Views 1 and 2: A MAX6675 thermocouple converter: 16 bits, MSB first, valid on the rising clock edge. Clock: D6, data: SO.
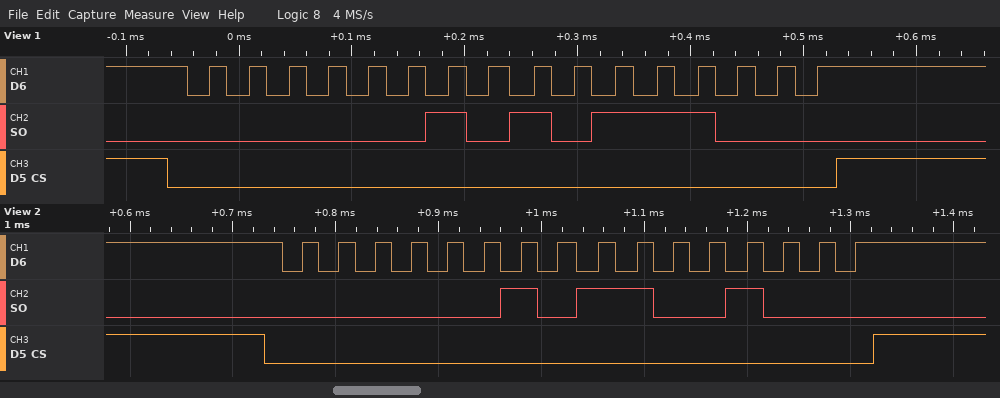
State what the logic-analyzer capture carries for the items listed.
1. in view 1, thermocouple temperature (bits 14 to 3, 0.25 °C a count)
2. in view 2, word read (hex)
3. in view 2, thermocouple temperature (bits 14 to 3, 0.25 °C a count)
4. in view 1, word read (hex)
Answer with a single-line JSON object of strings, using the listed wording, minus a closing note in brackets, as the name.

{"in view 1, thermocouple temperature": "21.75 °C", "in view 2, word read": "0x02C8", "in view 2, thermocouple temperature": "22.25 °C", "in view 1, word read": "0x02B8"}
